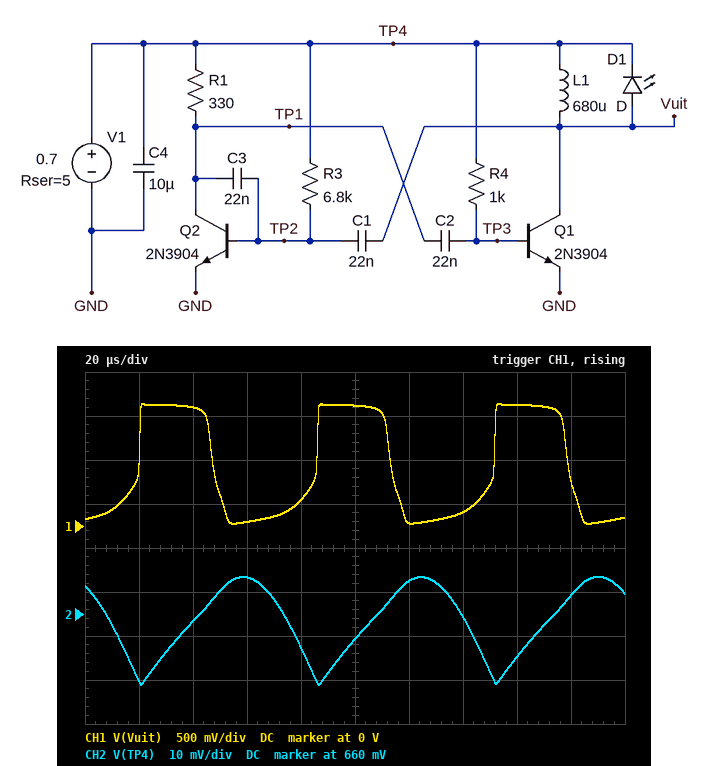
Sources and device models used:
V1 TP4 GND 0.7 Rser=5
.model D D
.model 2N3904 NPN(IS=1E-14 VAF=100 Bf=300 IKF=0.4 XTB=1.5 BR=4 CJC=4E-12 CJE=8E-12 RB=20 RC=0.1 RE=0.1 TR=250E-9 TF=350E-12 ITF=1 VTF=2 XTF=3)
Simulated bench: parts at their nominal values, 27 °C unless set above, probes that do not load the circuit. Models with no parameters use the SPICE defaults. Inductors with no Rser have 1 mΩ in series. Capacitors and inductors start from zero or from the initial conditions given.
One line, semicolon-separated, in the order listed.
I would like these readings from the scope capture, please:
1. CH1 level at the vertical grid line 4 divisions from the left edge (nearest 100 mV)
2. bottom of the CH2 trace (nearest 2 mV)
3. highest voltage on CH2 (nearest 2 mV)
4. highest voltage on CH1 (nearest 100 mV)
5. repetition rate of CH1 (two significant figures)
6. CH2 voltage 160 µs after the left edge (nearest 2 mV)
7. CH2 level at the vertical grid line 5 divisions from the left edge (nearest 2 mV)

300 mV; 644 mV; 668 mV; 1.4 V; 15 kHz; 650 mV; 654 mV
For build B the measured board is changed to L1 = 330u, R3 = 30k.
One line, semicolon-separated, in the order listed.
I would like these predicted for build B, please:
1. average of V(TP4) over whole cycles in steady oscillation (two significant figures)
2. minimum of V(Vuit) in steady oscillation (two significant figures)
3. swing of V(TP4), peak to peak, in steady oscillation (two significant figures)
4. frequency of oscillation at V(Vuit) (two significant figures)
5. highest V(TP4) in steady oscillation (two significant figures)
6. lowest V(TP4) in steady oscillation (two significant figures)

640 mV; 61 mV; 32 mV; 19 kHz; 650 mV; 620 mV
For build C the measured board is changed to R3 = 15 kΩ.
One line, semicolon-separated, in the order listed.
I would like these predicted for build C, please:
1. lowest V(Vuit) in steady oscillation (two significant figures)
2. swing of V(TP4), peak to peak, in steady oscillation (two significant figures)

28 mV; 26 mV
